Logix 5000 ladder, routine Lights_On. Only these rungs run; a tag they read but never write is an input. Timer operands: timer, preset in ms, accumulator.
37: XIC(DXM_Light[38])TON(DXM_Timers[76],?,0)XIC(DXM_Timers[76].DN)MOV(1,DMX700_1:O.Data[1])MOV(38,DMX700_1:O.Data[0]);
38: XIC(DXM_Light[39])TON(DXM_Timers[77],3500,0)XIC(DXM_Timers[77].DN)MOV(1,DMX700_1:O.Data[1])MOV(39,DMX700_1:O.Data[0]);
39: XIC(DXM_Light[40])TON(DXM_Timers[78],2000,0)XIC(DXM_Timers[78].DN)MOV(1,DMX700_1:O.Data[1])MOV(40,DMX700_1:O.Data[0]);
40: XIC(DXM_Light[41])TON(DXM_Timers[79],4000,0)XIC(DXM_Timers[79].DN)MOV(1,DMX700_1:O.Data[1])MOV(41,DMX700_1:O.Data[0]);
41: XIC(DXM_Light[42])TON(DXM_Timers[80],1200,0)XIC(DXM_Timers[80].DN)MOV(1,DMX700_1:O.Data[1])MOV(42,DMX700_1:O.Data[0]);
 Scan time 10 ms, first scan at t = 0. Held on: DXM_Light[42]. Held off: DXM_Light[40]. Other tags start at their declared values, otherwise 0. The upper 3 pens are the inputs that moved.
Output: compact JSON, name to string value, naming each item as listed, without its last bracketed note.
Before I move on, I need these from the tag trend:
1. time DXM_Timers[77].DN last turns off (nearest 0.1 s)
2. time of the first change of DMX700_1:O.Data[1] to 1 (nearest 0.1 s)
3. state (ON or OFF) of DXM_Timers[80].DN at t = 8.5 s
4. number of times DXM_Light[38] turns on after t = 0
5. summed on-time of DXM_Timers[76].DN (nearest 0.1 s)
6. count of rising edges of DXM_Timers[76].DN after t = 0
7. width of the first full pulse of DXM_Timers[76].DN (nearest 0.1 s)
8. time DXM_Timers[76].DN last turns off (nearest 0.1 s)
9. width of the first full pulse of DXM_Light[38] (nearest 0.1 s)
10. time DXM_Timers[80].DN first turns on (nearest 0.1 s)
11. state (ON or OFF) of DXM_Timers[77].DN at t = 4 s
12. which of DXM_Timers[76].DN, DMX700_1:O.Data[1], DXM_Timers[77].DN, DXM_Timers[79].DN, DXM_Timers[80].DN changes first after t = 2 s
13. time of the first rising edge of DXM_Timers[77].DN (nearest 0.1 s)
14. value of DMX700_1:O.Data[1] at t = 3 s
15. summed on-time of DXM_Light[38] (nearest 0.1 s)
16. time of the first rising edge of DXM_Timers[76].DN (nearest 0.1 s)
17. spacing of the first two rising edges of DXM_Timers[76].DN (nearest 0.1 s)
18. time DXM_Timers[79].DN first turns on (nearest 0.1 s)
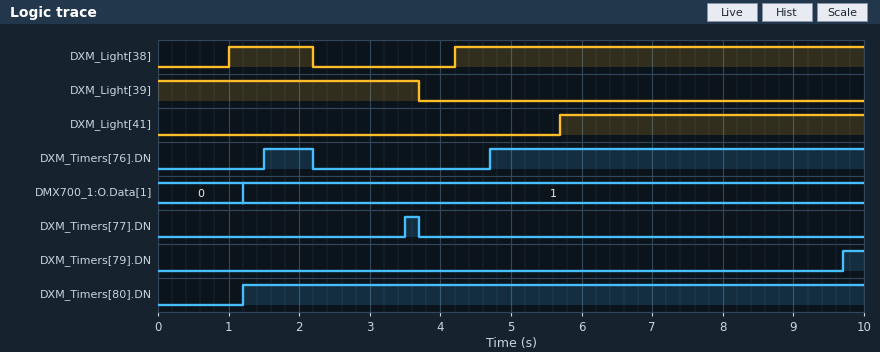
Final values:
{"time DXM_Timers[77].DN last turns off": "3.7 s", "time of the first change of DMX700_1:O.Data[1] to 1": "1.2 s", "state (ON or OFF) of DXM_Timers[80].DN at t = 8.5 s": "ON", "number of times DXM_Light[38] turns on after t = 0": "2", "summed on-time of DXM_Timers[76].DN": "6.0 s", "count of rising edges of DXM_Timers[76].DN after t = 0": "2", "width of the first full pulse of DXM_Timers[76].DN": "0.7 s", "time DXM_Timers[76].DN last turns off": "2.2 s", "width of the first full pulse of DXM_Light[38]": "1.2 s", "time DXM_Timers[80].DN first turns on": "1.2 s", "state (ON or OFF) of DXM_Timers[77].DN at t = 4 s": "OFF", "which of DXM_Timers[76].DN, DMX700_1:O.Data[1], DXM_Timers[77].DN, DXM_Timers[79].DN, DXM_Timers[80].DN changes first after t = 2 s": "DXM_Timers[76].DN", "time of the first rising edge of DXM_Timers[77].DN": "3.5 s", "value of DMX700_1:O.Data[1] at t = 3 s": "1", "summed on-time of DXM_Light[38]": "7.0 s", "time of the first rising edge of DXM_Timers[76].DN": "1.5 s", "spacing of the first two rising edges of DXM_Timers[76].DN": "3.2 s", "time DXM_Timers[79].DN first turns on": "9.7 s"}
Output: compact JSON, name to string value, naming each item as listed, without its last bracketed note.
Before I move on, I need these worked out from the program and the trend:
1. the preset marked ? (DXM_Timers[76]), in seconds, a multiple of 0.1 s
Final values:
{"the preset marked ? (DXM_Timers[76]), in seconds, a multiple of 0.1 s": "0.5 s"}
